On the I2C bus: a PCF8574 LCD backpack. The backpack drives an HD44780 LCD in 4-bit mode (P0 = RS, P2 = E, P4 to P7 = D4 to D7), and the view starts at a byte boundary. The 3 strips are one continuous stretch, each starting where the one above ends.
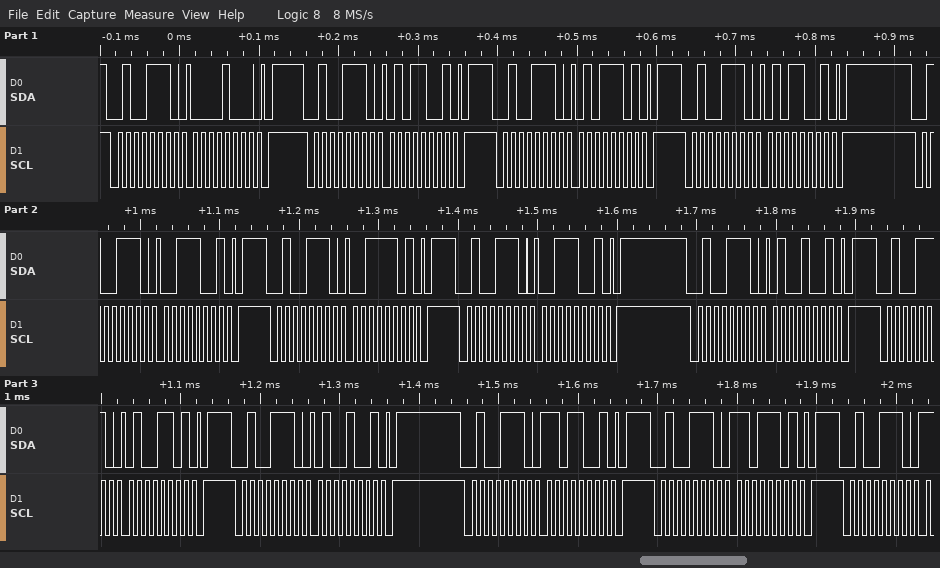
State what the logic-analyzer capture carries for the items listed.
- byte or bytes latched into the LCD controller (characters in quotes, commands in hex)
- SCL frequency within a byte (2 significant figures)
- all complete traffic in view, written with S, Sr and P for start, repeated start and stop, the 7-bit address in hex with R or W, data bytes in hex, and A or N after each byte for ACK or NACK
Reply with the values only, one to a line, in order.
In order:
'S'
100 kHz
S 27W A 08 A P S 27W A 59 A P S 27W A 5D A P S 27W A 59 A P S 27W A 39 A P S 27W A 3D A P S 27W A 39 A P S 27W A 49 A P S 27W A 4D A P S 27W A 49 A P S 27W A D9 A P S 27W A DD A P S 27W A
